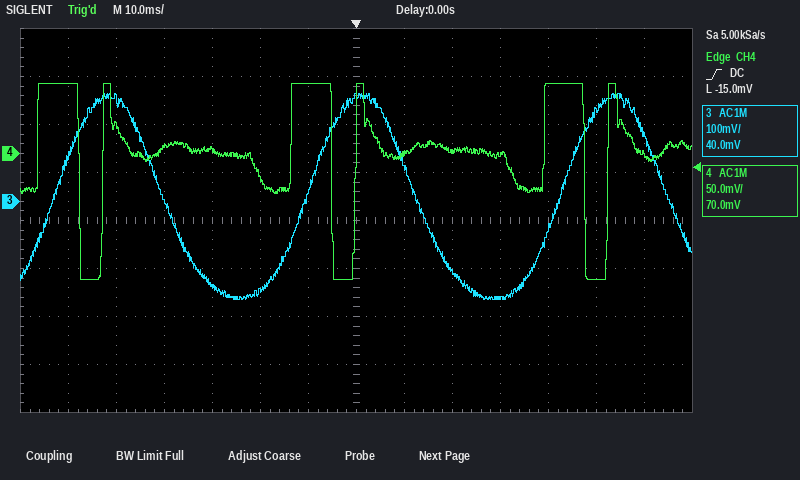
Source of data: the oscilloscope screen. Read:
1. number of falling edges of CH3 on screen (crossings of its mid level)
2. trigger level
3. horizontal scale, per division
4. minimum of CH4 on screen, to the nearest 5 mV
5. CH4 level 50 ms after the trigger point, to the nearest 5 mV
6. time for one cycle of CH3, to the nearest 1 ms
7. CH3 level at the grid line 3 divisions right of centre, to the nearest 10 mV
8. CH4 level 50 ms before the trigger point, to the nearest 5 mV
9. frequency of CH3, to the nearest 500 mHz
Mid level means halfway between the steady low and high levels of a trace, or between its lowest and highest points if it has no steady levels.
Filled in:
3
-15.0 mV
10 ms
-130 mV
-130 mV
53 ms
-200 mV
30 mV
19.0 Hz
